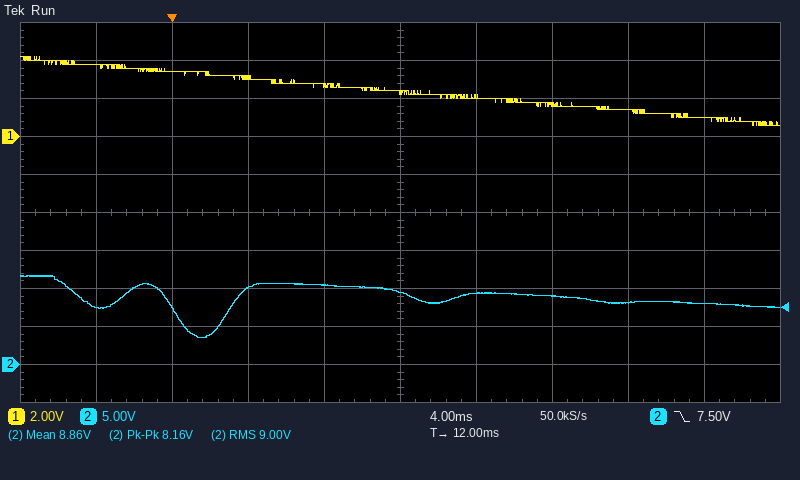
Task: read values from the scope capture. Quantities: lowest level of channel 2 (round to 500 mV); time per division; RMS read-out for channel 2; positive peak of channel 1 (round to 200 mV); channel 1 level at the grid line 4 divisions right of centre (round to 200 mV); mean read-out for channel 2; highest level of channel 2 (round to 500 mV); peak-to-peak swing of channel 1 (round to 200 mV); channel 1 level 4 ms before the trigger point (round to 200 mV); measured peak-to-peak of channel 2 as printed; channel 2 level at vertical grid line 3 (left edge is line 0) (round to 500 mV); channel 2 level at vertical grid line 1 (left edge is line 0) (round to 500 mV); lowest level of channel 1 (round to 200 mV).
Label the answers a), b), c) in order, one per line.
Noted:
a) 3.5 V
b) 4 ms
c) 9.00 V
d) 4.2 V
e) 1.0 V
f) 8.86 V
g) 11.5 V
h) 3.6 V
i) 3.8 V
j) 8.16 V
k) 10.0 V
l) 7.5 V
m) 600 mV
